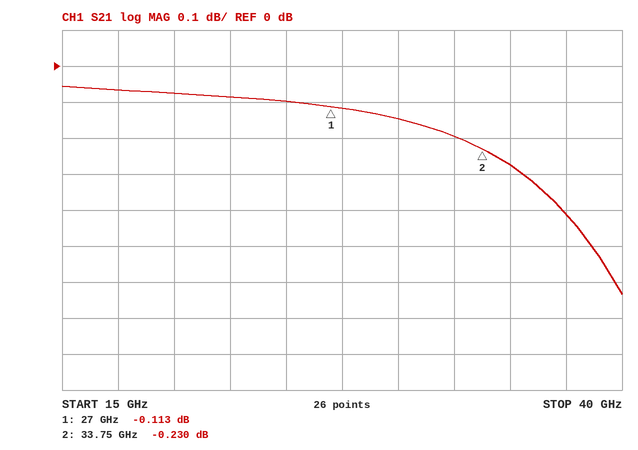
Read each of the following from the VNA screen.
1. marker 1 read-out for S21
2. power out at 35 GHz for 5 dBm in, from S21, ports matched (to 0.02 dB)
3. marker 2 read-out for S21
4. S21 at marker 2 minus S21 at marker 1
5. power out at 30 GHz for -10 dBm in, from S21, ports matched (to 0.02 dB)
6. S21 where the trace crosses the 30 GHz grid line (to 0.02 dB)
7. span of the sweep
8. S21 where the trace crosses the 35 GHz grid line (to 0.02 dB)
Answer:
-0.113 dB
4.72 dBm
-0.230 dB
-0.117 dB
-10.14 dBm
-0.14 dB
25 GHz
-0.28 dB
